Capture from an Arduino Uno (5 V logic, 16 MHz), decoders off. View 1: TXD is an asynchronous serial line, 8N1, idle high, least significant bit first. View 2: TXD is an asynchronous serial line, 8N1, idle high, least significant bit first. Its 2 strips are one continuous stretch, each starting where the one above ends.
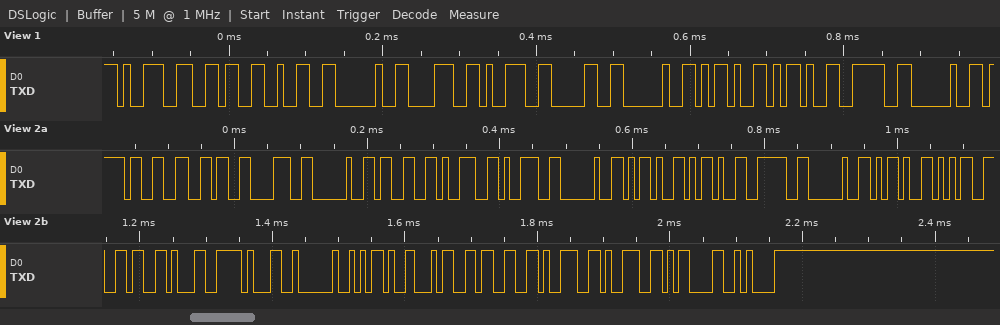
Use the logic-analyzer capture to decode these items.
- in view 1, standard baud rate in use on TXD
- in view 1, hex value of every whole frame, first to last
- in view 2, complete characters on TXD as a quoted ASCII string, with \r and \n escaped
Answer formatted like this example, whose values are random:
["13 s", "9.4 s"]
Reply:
["115200 baud", "39 36 32 20 38 39 30 20 2D 2D 3E 20", "\"368 399 --> -5611 -4399\\r\\n\""]
